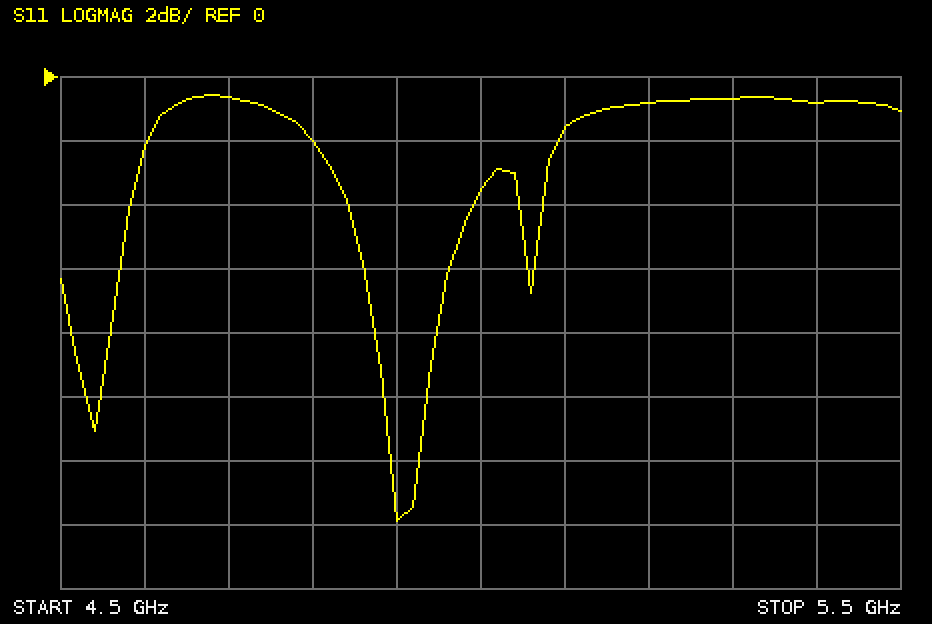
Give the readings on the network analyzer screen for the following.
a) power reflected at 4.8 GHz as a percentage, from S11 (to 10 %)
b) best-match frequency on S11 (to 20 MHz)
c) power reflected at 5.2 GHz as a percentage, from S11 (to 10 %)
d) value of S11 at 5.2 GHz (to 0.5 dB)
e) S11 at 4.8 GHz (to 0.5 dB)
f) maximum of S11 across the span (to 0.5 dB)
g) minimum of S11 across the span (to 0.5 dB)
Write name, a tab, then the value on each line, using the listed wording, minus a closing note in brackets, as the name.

power reflected at 4.8 GHz as a percentage, from S11	60 %
best-match frequency on S11	4.90 GHz
power reflected at 5.2 GHz as a percentage, from S11	80 %
value of S11 at 5.2 GHz	-1.0 dB
S11 at 4.8 GHz	-2.0 dB
maximum of S11 across the span	-0.5 dB
minimum of S11 across the span	-14.0 dB
